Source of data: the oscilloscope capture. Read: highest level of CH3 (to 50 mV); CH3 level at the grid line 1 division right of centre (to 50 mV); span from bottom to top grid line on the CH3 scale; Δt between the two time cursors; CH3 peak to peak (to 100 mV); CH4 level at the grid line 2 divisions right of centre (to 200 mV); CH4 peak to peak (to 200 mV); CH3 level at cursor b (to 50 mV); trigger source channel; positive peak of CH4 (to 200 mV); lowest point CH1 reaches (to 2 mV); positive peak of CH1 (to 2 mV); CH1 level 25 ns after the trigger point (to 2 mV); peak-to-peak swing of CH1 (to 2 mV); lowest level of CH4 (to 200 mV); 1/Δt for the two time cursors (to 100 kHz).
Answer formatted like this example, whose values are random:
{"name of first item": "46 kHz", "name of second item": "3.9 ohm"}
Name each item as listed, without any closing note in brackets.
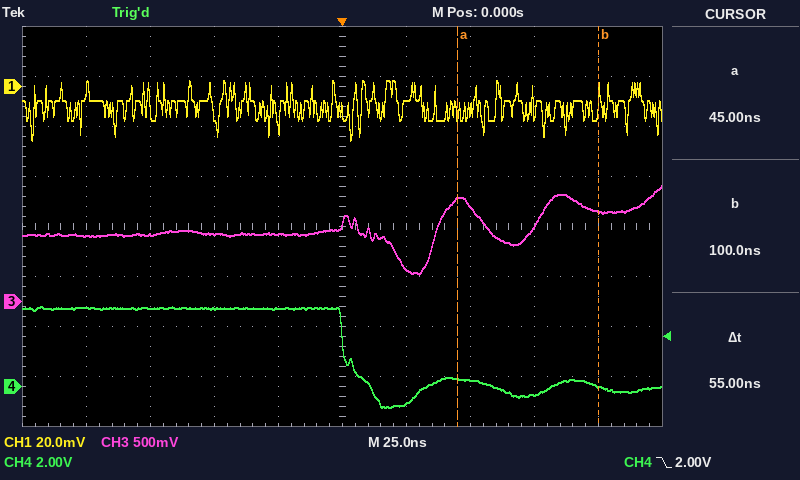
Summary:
{"highest level of CH3": "1.15 V", "CH3 level at the grid line 1 division right of centre": "350 mV", "span from bottom to top grid line on the CH3 scale": "4 V", "Δt between the two time cursors": "55 ns", "CH3 peak to peak": "900 mV", "CH4 level at the grid line 2 divisions right of centre": "200 mV", "CH4 peak to peak": "4.0 V", "CH3 level at cursor b": "900 mV", "trigger source channel": "CH4", "positive peak of CH4": "3.2 V", "lowest point CH1 reaches": "-22 mV", "positive peak of CH1": "2 mV", "CH1 level 25 ns after the trigger point": "-6 mV", "peak-to-peak swing of CH1": "24 mV", "lowest level of CH4": "-800 mV", "1/Δt for the two time cursors": "18.2 MHz"}
